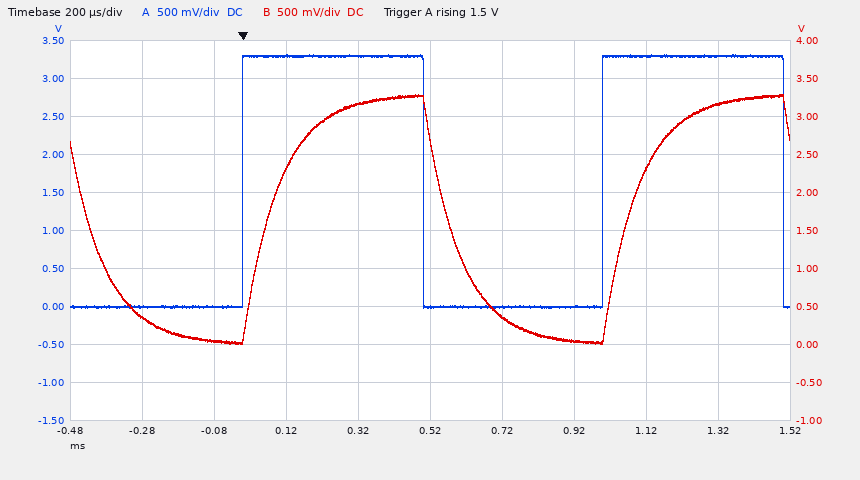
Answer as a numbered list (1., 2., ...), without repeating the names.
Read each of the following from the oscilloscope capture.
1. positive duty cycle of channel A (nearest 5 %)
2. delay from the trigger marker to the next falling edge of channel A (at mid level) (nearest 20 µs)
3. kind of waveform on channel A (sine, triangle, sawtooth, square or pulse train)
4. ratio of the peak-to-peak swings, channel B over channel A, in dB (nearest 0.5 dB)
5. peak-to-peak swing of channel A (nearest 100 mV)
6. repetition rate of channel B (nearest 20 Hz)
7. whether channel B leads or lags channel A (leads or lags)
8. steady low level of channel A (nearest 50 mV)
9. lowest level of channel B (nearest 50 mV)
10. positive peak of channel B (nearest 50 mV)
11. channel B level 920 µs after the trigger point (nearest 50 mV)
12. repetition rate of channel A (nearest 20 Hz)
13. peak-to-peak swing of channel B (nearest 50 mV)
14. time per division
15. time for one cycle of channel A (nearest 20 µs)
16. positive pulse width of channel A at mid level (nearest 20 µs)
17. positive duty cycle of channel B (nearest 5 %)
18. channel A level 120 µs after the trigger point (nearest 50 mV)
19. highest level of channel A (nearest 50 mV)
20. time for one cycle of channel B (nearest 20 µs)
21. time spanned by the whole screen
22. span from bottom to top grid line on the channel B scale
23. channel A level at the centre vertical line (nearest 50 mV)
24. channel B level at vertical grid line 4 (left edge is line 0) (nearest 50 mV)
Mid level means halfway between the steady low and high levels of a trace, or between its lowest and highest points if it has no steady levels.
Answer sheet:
1. 50 %
2. 500 µs
3. square
4. 0.0 dB
5. 3.30 V
6. 1.00 kHz
7. lags
8. 0 mV
9. 0 mV
10. 3.30 V
11. 50 mV
12. 1.00 kHz
13. 3.30 V
14. 200 µs
15. 1.00 ms
16. 500 µs
17. 50 %
18. 3.30 V
19. 3.30 V
20. 1.00 ms
21. 2 ms
22. 5 V
23. 0 mV
24. 3.15 V
